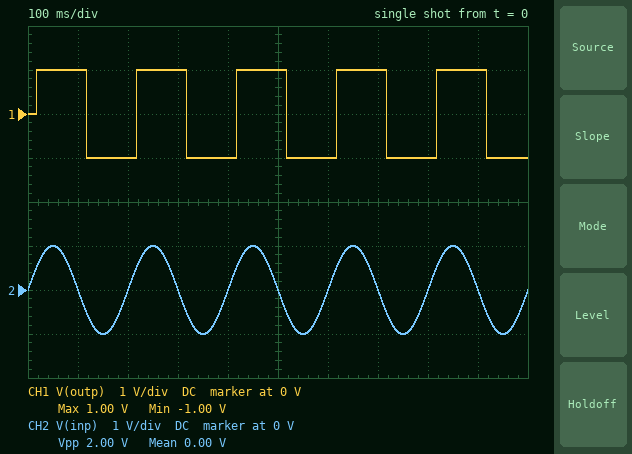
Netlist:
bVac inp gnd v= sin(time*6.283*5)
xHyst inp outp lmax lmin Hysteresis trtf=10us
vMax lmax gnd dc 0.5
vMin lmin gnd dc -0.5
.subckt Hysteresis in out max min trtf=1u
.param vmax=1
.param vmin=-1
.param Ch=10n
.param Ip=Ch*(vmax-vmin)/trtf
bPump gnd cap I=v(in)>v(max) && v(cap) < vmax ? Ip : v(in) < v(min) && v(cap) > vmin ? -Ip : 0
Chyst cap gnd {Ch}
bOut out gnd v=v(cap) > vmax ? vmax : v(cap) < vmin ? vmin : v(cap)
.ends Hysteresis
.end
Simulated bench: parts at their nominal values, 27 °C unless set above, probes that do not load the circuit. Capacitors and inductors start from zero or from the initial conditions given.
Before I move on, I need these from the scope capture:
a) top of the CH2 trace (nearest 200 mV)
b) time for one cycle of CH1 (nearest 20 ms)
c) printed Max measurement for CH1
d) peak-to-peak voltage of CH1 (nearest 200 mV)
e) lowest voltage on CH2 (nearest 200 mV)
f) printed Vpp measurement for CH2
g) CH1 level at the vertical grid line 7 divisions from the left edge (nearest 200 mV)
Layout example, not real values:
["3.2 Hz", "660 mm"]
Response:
["1.0 V", "200 ms", "1.00 V", "2.0 V", "-1.0 V", "2.00 V", "1.0 V"]
